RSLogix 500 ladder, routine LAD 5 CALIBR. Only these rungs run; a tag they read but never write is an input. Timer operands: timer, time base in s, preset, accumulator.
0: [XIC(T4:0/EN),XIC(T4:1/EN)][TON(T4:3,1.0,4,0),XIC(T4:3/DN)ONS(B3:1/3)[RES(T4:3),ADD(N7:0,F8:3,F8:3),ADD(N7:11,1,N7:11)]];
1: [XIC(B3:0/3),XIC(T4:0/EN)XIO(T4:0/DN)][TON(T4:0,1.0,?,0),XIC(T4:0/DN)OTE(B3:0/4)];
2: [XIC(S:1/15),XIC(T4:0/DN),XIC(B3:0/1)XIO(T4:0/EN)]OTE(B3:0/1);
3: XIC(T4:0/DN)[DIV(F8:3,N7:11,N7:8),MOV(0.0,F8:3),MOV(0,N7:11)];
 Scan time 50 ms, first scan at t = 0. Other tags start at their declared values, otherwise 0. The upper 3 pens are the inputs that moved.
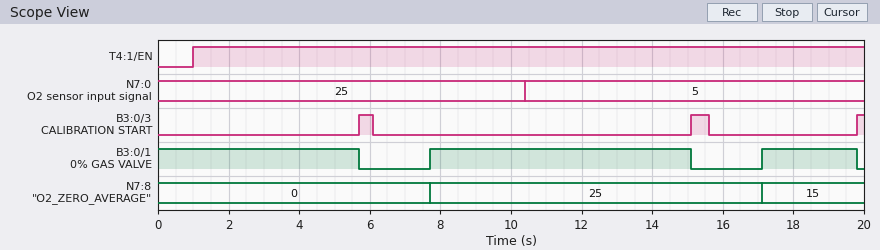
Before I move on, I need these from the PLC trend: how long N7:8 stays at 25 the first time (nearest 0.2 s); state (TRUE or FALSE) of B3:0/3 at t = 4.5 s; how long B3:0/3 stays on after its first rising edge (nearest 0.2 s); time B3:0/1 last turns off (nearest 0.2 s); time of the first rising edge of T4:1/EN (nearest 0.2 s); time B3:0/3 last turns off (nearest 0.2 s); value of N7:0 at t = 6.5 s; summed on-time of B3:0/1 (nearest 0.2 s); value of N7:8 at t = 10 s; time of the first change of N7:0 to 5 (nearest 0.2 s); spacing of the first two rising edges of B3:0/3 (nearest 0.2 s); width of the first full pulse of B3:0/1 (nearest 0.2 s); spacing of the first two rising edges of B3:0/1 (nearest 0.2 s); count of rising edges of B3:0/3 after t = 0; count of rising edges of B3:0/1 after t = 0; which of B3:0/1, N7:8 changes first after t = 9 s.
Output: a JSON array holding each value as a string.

["9.4 s", "FALSE", "0.4 s", "19.8 s", "1.0 s", "15.6 s", "25", "15.8 s", "25", "10.4 s", "9.4 s", "7.4 s", "9.4 s", "3", "2", "B3:0/1"]
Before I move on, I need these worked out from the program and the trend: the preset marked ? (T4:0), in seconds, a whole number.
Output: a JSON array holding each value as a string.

["2 s"]
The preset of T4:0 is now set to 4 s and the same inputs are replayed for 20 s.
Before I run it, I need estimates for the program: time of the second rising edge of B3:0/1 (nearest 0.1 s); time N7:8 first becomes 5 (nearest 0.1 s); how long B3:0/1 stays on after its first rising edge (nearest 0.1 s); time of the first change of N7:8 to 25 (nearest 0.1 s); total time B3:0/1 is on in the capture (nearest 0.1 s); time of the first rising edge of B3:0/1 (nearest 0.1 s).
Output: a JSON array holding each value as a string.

["19.1 s", "19.1 s", "5.4 s", "9.7 s", "11.8 s", "9.7 s"]
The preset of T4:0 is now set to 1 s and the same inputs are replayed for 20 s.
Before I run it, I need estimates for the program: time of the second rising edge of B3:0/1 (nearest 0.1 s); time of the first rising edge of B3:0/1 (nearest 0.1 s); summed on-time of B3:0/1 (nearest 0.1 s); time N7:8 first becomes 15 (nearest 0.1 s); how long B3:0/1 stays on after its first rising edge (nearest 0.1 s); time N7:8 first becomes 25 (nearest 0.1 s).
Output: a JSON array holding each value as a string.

["16.1 s", "6.7 s", "17.8 s", "16.1 s", "8.4 s", "6.7 s"]
